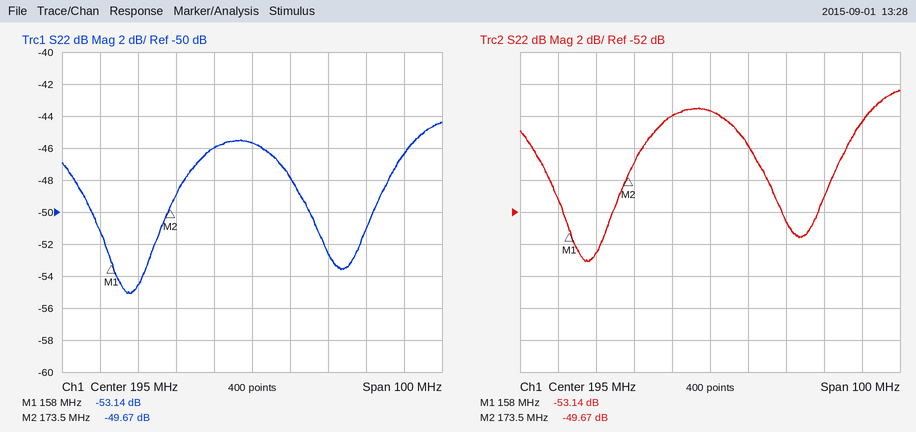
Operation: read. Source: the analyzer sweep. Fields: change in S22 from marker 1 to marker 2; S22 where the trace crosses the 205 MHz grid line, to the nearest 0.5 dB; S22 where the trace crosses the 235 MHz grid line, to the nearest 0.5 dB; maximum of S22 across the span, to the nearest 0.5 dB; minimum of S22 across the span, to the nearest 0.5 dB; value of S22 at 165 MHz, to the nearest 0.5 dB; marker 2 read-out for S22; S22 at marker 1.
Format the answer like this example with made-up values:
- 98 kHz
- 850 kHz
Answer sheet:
- 3.47 dB
- -48.0 dB
- -46.5 dB
- -44.5 dB
- -55.0 dB
- -54.5 dB
- -49.67 dB
- -53.14 dB
